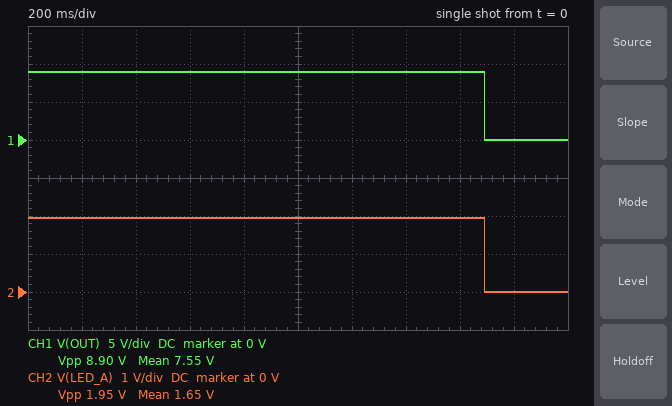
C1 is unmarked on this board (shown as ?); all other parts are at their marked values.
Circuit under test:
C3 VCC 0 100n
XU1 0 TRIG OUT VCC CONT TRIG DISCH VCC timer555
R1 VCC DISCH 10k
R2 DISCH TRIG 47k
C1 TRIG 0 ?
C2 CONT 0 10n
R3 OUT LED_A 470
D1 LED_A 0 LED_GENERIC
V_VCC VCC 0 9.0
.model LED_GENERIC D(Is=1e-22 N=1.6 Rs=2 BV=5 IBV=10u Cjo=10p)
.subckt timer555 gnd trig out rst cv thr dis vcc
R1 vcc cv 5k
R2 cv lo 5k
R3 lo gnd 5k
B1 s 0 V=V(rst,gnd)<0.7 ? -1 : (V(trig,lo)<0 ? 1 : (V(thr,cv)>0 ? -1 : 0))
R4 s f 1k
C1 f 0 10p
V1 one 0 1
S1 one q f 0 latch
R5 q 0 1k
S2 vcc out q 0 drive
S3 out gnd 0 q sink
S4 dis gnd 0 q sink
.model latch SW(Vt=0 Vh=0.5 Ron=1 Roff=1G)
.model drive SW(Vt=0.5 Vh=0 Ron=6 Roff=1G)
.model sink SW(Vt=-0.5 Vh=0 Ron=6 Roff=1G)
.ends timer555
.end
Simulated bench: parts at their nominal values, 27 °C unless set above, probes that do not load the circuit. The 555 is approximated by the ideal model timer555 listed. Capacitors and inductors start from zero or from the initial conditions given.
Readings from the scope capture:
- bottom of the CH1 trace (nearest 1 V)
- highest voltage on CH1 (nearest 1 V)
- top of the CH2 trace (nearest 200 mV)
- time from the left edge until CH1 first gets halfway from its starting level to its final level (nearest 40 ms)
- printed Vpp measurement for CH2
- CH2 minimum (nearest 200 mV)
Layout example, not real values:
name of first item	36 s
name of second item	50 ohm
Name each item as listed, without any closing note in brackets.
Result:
bottom of the CH1 trace	0 V
highest voltage on CH1	9 V
top of the CH2 trace	2.0 V
time from the left edge until CH1 first gets halfway from its starting level to its final level	1.68 s
printed Vpp measurement for CH2	1.95 V
CH2 minimum	0 V
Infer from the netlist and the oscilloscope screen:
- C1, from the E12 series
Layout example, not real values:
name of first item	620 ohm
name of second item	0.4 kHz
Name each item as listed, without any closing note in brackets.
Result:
C1, from the E12 series	27 µF
